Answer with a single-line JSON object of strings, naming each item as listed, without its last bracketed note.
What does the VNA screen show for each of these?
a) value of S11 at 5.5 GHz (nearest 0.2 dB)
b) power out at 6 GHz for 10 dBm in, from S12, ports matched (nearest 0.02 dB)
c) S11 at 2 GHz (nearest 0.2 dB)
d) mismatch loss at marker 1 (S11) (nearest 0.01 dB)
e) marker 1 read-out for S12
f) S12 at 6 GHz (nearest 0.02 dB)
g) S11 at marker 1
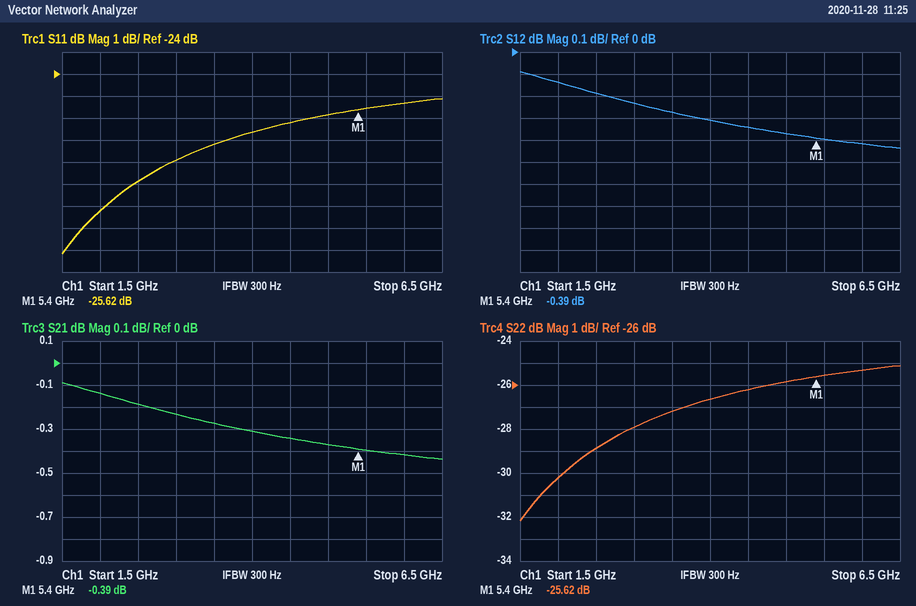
{"value of S11 at 5.5 GHz": "-25.6 dB", "power out at 6 GHz for 10 dBm in, from S12, ports matched": "9.58 dBm", "S11 at 2 GHz": "-30.2 dB", "mismatch loss at marker 1 (S11)": "0.01 dB", "marker 1 read-out for S12": "-0.39 dB", "S12 at 6 GHz": "-0.42 dB", "S11 at marker 1": "-25.62 dB"}
